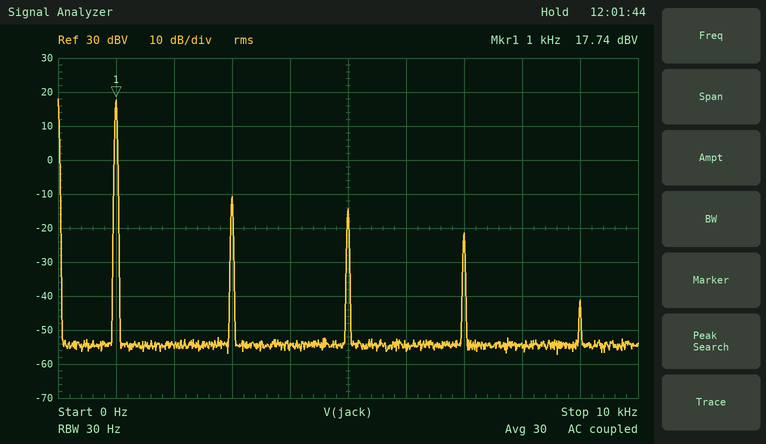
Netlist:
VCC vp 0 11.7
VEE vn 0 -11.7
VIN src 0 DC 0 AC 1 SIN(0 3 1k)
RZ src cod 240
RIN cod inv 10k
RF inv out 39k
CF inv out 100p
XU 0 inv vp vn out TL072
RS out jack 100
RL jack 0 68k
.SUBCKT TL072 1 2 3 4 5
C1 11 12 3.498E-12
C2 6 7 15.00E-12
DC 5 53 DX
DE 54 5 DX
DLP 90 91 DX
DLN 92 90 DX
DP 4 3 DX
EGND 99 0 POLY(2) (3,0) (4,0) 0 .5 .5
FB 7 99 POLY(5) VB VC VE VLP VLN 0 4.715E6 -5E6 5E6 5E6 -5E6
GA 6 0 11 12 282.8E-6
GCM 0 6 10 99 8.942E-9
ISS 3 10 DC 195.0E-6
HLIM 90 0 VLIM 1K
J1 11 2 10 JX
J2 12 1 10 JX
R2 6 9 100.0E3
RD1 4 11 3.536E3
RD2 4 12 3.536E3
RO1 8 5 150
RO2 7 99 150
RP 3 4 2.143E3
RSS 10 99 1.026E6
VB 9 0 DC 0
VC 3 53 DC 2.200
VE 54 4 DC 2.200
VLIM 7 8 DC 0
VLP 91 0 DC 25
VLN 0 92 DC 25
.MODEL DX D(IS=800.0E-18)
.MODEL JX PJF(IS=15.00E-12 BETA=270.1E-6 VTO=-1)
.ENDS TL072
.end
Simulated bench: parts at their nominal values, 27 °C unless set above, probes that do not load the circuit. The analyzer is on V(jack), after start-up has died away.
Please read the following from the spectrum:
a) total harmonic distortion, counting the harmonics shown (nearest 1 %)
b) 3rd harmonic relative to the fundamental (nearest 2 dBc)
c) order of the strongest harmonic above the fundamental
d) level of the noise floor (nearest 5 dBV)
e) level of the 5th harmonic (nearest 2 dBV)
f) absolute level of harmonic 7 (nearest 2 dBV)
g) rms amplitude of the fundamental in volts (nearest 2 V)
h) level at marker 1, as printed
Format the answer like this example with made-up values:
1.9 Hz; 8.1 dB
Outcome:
5 %; -28 dBc; 3; -55 dBV; -14 dBV; -22 dBV; 8 V; 17.74 dBV
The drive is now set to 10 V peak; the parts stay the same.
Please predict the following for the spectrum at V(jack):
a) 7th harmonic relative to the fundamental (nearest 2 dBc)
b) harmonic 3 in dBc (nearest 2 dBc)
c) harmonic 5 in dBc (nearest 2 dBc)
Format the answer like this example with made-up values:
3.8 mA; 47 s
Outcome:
-22 dBc; -10 dBc; -16 dBc
